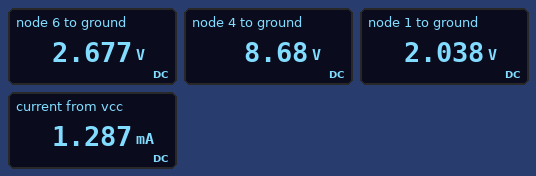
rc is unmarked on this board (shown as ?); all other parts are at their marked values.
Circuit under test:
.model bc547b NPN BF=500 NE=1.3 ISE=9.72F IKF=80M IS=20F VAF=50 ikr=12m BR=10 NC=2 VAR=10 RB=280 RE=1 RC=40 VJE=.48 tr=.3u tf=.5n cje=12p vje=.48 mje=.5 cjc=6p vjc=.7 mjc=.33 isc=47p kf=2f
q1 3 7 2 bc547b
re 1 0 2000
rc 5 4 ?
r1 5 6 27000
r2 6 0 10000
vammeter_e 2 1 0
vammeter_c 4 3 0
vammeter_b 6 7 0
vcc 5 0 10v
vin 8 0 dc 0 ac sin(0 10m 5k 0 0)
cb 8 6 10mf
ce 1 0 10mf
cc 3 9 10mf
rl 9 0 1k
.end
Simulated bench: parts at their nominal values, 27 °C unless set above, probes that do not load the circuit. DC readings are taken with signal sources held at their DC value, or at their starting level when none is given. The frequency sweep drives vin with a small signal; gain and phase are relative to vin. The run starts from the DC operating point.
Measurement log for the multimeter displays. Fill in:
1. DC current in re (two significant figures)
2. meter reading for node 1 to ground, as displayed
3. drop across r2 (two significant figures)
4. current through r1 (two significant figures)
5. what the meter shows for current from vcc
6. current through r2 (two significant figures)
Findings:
1.0 mA
2.038 V
2.7 V
270 µA
1.287 mA
270 µA
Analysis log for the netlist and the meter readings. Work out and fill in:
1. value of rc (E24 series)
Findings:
1.3 kΩ
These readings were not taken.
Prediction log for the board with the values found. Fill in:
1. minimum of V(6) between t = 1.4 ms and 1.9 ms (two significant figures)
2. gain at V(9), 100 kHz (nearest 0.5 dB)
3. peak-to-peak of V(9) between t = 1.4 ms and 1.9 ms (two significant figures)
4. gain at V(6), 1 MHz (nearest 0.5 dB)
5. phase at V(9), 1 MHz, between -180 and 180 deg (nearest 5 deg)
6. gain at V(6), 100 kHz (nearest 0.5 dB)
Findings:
2.7 V
26.0 dB
410 mV
0 dB
170 deg
0 dB
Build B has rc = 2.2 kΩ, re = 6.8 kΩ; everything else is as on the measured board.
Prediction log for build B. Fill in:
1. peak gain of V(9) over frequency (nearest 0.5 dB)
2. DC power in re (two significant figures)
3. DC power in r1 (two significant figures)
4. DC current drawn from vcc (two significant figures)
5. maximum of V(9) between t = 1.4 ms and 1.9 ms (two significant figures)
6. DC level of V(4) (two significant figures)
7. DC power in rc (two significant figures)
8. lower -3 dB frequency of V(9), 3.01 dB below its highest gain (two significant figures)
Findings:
18.0 dB
640 µW
2.0 mW
580 µA
66 mV
9.3 V
210 µW
190 mHz
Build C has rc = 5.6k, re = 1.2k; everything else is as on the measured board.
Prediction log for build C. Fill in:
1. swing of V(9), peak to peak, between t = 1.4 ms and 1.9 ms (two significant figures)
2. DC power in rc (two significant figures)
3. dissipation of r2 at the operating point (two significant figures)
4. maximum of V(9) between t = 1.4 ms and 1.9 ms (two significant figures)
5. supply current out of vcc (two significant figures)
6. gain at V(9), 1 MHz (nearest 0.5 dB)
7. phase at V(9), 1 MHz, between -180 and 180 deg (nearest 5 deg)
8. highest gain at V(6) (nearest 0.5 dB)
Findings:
43 mV
12 mW
600 µW
31 mV
1.7 mA
-16.0 dB
75 deg
0 dB
